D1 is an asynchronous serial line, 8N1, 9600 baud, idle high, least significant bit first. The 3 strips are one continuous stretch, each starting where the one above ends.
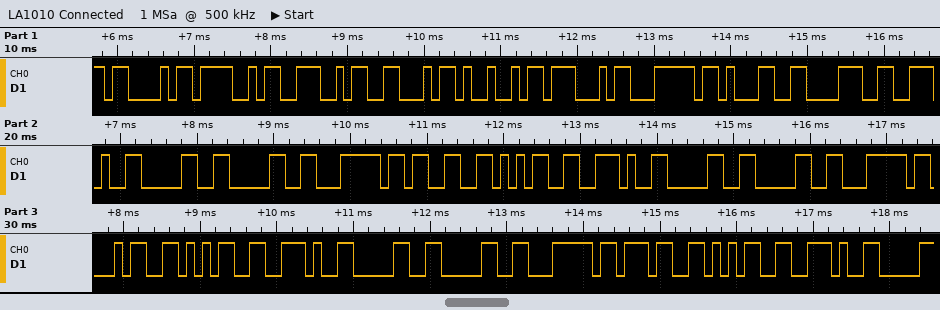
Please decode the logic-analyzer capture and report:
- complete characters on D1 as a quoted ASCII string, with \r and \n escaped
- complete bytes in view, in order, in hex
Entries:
"CONFIG|18.00|35.00|45.00|75."
43 4F 4E 46 49 47 7C 31 38 2E 30 30 7C 33 35 2E 30 30 7C 34 35 2E 30 30 7C 37 35 2E
